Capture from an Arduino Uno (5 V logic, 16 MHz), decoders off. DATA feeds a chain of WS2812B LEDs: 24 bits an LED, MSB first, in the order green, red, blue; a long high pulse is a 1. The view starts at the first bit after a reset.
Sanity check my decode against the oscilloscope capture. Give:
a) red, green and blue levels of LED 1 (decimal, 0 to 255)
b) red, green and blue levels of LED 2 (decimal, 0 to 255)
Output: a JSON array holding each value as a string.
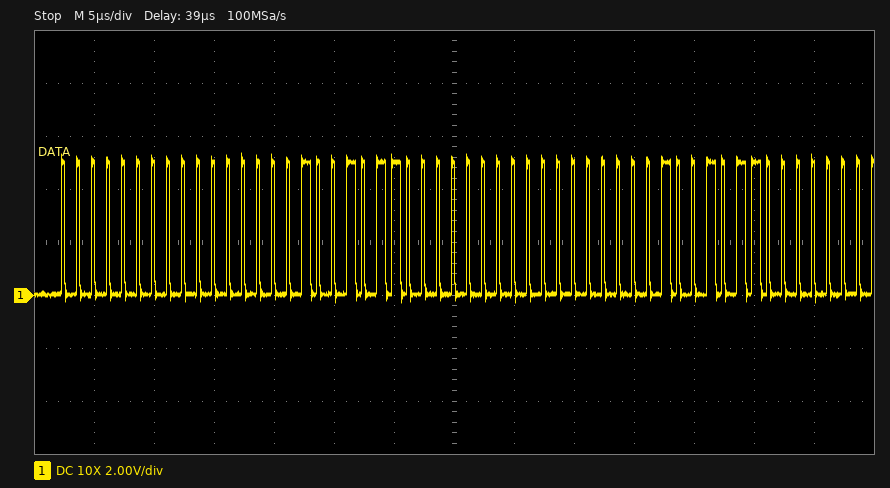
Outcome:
["0, 0, 150", "0, 0, 150"]
